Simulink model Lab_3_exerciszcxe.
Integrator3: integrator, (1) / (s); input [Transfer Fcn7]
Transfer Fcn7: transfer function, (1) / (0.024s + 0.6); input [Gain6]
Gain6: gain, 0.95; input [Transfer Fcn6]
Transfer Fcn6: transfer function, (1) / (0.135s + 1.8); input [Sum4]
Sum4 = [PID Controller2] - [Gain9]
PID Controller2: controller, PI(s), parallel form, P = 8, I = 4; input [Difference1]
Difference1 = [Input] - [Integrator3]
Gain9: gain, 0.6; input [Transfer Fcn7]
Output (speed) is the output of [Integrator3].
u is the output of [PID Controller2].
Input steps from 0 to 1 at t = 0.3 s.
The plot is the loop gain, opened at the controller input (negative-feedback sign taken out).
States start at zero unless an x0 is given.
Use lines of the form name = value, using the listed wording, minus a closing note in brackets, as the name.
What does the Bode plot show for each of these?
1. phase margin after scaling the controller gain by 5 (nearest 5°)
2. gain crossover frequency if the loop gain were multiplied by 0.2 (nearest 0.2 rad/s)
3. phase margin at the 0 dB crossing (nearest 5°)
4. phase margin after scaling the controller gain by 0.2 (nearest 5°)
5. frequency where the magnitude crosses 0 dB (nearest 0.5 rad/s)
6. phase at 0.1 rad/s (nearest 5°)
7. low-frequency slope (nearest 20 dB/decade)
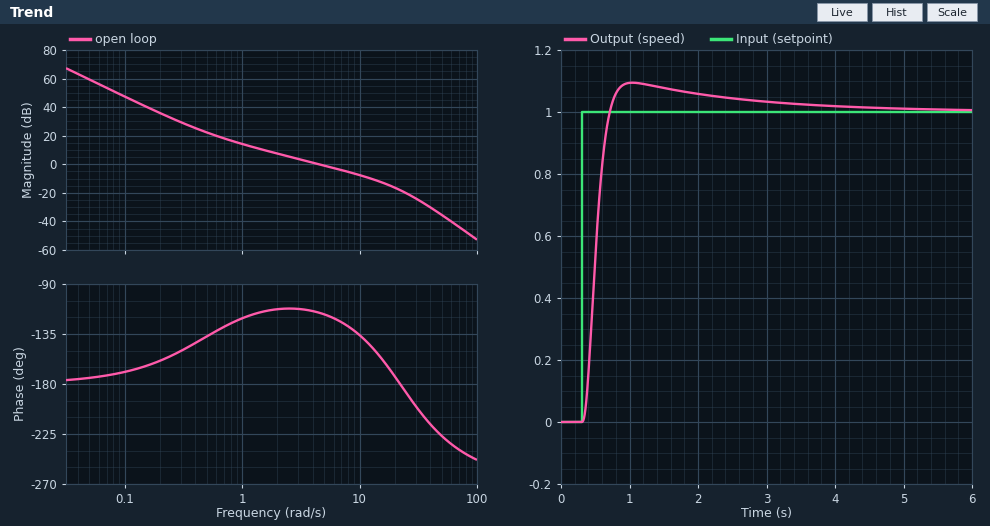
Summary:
phase margin after scaling the controller gain by 5 = 15°
gain crossover frequency if the loop gain were multiplied by 0.2 = 1.0 rad/s
phase margin at the 0 dB crossing = 65°
phase margin after scaling the controller gain by 0.2 = 60°
frequency where the magnitude crosses 0 dB = 4.5 rad/s
phase at 0.1 rad/s = -170°
low-frequency slope = -40 dB/decade
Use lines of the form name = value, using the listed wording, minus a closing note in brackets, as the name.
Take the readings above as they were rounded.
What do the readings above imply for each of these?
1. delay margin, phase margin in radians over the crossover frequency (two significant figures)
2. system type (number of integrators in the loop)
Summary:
delay margin, phase margin in radians over the crossover frequency = 0.25 s
system type = 2
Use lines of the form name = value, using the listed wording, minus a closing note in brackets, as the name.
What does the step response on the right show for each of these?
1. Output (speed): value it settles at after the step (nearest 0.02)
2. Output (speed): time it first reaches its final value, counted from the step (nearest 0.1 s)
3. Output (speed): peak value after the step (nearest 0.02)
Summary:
Output (speed): value it settles at after the step = 1.00
Output (speed): time it first reaches its final value, counted from the step = 0.4 s
Output (speed): peak value after the step = 1.10
